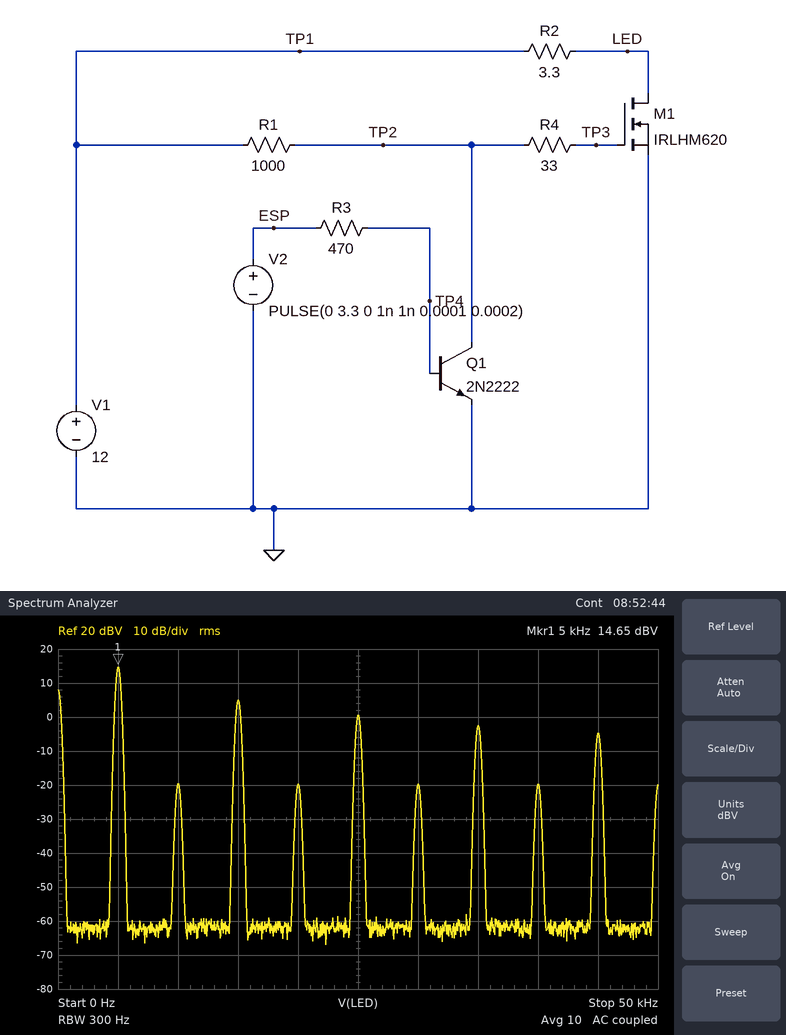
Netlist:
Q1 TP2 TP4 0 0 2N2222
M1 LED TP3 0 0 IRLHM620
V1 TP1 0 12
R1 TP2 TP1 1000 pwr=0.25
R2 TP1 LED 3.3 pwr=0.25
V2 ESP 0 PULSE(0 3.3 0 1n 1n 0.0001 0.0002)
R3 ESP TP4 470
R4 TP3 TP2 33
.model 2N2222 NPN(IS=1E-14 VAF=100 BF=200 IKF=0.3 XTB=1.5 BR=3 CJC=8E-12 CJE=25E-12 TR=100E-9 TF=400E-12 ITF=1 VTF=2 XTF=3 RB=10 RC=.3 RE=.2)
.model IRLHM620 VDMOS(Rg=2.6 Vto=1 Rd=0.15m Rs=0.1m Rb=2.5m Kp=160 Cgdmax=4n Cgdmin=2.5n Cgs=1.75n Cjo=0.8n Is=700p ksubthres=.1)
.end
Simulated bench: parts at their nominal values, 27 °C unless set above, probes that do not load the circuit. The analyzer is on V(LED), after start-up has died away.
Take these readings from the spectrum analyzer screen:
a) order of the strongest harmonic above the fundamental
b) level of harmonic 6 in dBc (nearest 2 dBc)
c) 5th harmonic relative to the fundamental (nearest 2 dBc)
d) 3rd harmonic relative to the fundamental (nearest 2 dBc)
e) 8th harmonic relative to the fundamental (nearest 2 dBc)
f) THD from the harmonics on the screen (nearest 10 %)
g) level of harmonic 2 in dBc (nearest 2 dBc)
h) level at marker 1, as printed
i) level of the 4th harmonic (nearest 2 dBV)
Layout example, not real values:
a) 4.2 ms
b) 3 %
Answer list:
a) 3
b) -34 dBc
c) -14 dBc
d) -10 dBc
e) -34 dBc
f) 40 %
g) -34 dBc
h) 14.65 dBV
i) -20 dBV
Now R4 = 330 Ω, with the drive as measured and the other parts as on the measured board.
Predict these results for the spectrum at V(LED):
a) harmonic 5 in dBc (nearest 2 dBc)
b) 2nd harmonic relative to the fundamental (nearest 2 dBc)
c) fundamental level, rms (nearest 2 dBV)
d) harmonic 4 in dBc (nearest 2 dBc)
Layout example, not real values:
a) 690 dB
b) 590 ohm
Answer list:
a) -16 dBc
b) -20 dBc
c) 14 dBV
d) -20 dBc
